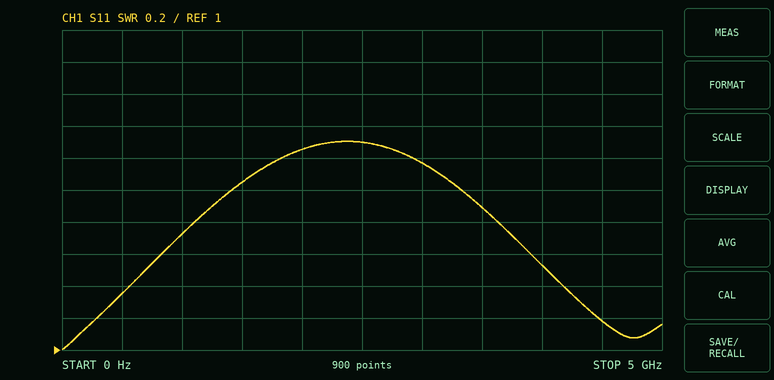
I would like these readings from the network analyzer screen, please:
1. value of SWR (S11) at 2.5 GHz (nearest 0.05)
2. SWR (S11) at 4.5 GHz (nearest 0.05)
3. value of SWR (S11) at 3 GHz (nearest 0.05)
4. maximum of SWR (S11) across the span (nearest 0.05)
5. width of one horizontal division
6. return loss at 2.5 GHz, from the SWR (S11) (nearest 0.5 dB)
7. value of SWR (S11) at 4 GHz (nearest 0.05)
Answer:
2.30
1.20
2.15
2.30
500 MHz
8.0 dB
1.55
